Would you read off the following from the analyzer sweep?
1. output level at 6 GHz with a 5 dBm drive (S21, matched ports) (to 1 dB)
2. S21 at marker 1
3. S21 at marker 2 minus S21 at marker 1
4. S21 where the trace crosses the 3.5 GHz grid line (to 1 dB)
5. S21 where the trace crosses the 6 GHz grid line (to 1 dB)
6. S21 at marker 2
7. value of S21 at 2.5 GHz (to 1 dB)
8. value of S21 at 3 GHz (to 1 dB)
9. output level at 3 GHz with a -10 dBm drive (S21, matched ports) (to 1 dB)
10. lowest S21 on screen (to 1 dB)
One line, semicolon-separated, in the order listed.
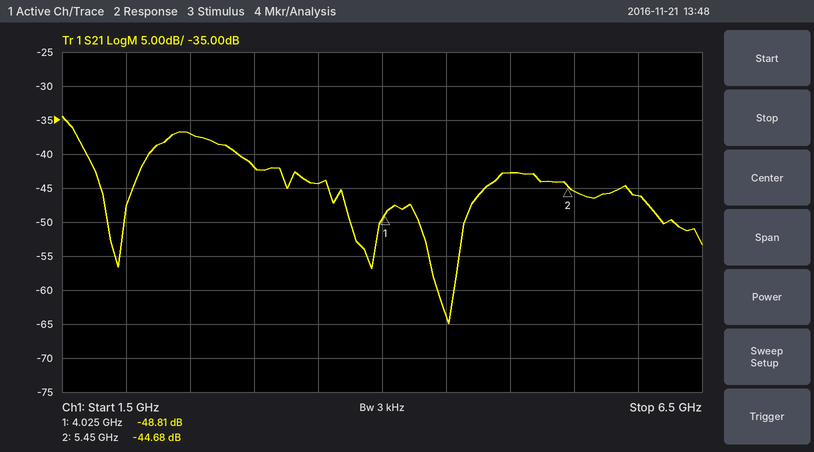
-41 dBm; -48.81 dB; 4.13 dB; -44 dB; -46 dB; -44.68 dB; -37 dB; -42 dB; -52 dBm; -65 dB
